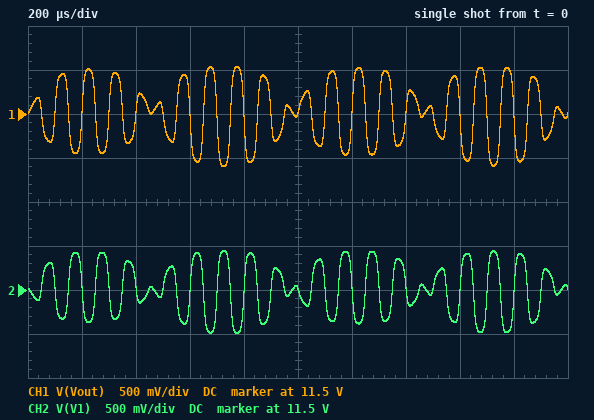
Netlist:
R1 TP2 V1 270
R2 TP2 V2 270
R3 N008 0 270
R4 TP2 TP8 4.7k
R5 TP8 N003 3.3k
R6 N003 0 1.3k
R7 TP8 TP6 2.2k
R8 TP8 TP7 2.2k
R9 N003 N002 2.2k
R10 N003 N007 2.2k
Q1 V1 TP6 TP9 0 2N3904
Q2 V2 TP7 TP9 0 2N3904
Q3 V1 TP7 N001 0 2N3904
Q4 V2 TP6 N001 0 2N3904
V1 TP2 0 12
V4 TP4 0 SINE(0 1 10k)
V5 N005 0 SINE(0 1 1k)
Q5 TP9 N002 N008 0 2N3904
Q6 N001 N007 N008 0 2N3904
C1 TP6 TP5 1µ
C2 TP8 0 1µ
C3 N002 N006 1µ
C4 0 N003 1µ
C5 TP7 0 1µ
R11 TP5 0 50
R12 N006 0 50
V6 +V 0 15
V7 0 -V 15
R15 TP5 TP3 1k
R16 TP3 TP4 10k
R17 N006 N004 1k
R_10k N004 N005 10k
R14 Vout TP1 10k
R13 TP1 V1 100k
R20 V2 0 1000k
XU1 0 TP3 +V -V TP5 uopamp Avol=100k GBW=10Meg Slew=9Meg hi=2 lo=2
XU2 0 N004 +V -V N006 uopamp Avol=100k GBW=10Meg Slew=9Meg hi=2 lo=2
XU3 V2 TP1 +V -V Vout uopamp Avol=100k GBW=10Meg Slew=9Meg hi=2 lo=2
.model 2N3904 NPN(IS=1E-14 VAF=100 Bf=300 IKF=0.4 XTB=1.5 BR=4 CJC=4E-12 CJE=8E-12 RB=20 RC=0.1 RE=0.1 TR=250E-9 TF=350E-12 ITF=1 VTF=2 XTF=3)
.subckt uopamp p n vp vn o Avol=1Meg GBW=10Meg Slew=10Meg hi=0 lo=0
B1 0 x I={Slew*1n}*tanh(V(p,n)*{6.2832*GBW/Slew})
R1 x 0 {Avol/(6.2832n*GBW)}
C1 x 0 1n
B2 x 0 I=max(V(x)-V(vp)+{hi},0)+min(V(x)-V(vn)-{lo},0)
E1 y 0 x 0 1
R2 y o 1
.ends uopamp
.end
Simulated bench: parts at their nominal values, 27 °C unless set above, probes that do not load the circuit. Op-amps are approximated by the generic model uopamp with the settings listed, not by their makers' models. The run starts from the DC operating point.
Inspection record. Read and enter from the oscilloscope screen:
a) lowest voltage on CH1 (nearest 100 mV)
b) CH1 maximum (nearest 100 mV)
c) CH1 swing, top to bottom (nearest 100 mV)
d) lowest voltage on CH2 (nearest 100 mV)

10.9 V
12.0 V
1.1 V
11.0 V
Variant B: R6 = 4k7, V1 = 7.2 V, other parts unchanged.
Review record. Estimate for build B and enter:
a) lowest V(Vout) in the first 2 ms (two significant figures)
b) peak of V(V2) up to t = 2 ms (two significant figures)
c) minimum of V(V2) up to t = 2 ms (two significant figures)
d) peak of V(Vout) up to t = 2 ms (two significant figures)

5.2 V
7.1 V
5.4 V
7.2 V
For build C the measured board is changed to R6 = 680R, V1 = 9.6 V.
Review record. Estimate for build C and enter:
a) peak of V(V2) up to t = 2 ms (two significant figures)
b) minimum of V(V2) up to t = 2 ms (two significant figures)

9.6 V
9.4 V
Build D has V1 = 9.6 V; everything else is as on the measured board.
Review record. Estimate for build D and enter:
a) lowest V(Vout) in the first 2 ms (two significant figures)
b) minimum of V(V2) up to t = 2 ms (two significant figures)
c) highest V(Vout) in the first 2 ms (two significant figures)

8.8 V
8.9 V
9.6 V
